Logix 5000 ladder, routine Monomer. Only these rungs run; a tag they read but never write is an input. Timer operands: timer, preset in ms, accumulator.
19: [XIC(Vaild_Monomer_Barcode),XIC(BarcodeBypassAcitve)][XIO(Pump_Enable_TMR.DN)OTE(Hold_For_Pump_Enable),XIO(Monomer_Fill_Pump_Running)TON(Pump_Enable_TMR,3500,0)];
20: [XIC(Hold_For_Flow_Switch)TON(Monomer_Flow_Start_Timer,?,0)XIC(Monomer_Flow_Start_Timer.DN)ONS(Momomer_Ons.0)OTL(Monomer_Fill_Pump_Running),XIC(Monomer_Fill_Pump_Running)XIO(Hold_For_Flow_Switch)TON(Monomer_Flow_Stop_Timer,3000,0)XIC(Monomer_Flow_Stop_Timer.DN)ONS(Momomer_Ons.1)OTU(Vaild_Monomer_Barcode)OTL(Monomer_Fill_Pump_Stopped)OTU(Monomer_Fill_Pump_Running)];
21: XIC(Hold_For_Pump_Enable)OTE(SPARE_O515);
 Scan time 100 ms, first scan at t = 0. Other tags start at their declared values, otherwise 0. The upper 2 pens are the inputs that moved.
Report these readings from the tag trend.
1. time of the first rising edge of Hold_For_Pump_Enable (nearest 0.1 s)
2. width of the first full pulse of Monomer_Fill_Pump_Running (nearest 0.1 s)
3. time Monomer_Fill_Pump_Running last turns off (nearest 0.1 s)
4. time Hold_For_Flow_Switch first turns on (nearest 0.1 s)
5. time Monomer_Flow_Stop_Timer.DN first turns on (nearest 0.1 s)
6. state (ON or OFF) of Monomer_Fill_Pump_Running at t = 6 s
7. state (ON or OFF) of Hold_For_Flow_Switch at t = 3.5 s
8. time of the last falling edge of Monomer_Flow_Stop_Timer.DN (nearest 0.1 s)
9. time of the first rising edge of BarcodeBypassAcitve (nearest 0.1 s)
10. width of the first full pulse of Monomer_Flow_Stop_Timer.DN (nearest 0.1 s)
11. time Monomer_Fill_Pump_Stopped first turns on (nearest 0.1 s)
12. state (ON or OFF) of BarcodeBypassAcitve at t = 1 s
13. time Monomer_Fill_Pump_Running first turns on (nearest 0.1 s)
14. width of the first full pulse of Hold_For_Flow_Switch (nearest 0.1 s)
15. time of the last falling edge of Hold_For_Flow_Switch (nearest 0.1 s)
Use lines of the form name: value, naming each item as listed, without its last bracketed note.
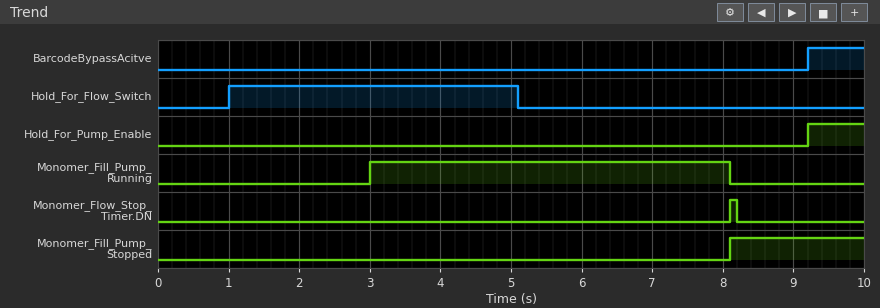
time of the first rising edge of Hold_For_Pump_Enable: 9.2 s
width of the first full pulse of Monomer_Fill_Pump_Running: 5.1 s
time Monomer_Fill_Pump_Running last turns off: 8.1 s
time Hold_For_Flow_Switch first turns on: 1.0 s
time Monomer_Flow_Stop_Timer.DN first turns on: 8.1 s
state (ON or OFF) of Monomer_Fill_Pump_Running at t = 6 s: ON
state (ON or OFF) of Hold_For_Flow_Switch at t = 3.5 s: ON
time of the last falling edge of Monomer_Flow_Stop_Timer.DN: 8.2 s
time of the first rising edge of BarcodeBypassAcitve: 9.2 s
width of the first full pulse of Monomer_Flow_Stop_Timer.DN: 0.1 s
time Monomer_Fill_Pump_Stopped first turns on: 8.1 s
state (ON or OFF) of BarcodeBypassAcitve at t = 1 s: OFF
time Monomer_Fill_Pump_Running first turns on: 3.0 s
width of the first full pulse of Hold_For_Flow_Switch: 4.1 s
time of the last falling edge of Hold_For_Flow_Switch: 5.1 s
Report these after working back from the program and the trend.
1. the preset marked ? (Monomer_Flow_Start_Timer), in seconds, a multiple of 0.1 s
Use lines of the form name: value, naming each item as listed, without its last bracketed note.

the preset marked ? (Monomer_Flow_Start_Timer), in seconds, a multiple of 0.1 s: 2.0 s
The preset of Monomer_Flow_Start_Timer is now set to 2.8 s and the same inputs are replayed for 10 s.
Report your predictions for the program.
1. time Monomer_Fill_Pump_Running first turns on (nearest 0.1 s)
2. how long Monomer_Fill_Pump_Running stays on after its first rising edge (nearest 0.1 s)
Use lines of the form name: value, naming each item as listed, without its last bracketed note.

time Monomer_Fill_Pump_Running first turns on: 3.8 s
how long Monomer_Fill_Pump_Running stays on after its first rising edge: 4.3 s
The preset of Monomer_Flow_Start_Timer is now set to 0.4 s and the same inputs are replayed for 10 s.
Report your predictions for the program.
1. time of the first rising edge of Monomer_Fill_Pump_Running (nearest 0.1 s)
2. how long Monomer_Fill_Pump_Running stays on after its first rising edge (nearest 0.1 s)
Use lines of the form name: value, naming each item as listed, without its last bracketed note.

time of the first rising edge of Monomer_Fill_Pump_Running: 1.4 s
how long Monomer_Fill_Pump_Running stays on after its first rising edge: 6.7 s
